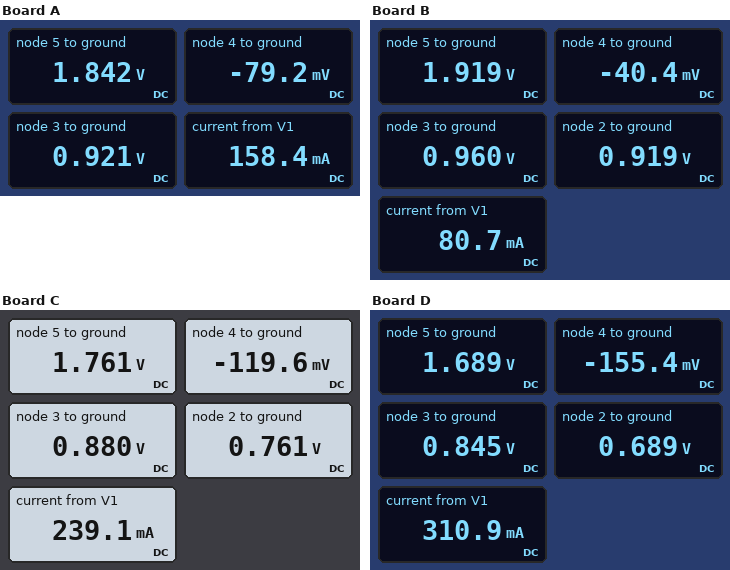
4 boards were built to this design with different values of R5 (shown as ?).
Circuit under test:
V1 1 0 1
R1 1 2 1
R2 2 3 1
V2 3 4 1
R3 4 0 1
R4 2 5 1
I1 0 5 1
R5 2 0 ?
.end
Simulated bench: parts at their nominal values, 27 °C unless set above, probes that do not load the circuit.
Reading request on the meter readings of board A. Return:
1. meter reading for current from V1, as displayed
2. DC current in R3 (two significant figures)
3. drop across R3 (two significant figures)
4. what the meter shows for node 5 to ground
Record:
158.4 mA
79 mA
79 mV
1.842 V
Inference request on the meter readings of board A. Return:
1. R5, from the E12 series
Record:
0.68 Ω
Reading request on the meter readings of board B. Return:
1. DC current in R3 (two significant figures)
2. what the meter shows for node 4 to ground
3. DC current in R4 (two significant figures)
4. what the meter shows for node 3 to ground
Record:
40 mA
-40.4 mV
1.0 A
0.960 V
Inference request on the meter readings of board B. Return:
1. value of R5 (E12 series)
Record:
0.82 Ω
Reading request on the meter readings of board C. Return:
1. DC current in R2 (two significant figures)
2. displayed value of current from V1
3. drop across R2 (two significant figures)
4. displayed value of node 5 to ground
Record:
120 mA
239.1 mA
120 mV
1.761 V
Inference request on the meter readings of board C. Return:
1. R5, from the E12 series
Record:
0.56 Ω
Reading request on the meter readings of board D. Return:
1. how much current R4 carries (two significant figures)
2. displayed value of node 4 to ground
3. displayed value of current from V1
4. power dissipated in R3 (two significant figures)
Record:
1.0 A
-155.4 mV
310.9 mA
24 mW
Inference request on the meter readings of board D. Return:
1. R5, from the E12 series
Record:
0.47 Ω
